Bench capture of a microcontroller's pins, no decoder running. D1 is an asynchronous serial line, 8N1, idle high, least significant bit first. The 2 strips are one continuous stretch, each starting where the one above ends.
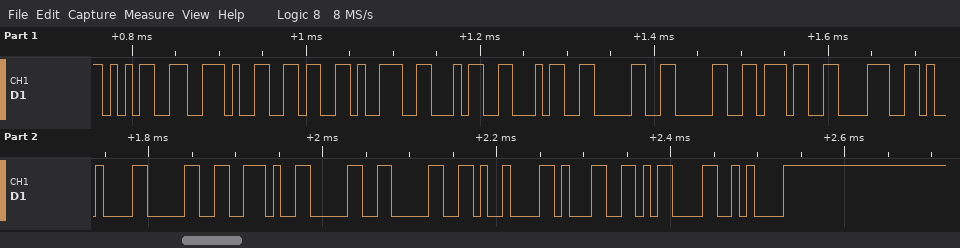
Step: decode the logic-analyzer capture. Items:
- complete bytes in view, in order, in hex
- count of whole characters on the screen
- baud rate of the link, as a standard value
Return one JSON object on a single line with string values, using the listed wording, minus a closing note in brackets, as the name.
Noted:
{"complete bytes in view, in order, in hex": "0x35 0x2E 0x36 0x39 0x34 0x34 0x30 0x30 0x37 0x38 0x09 0x30 0x2E 0x30 0x30 0x09 0x31 0x0D 0x0A", "count of whole characters on the screen": "19", "baud rate of the link, as a standard value": "115200 baud"}
